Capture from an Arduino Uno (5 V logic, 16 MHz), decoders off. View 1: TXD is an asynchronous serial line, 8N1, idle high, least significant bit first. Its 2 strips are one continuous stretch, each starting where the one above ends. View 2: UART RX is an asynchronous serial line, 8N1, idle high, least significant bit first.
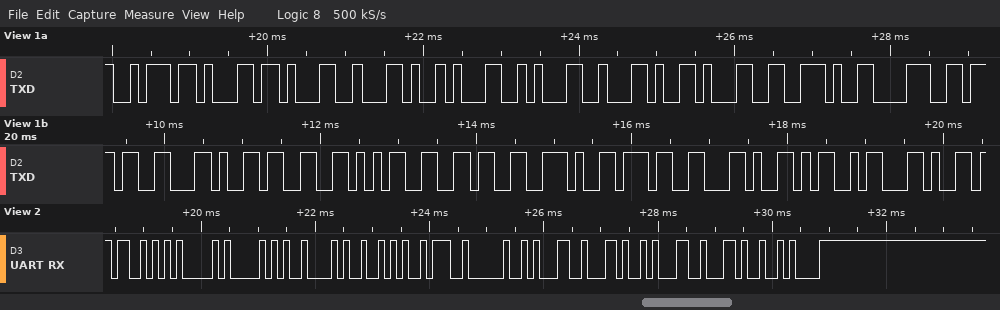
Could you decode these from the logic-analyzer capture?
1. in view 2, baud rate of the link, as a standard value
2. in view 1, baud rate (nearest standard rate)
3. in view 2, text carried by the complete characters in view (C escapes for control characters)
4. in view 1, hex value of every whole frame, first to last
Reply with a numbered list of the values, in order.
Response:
1. 9600 baud
2. 9600 baud
3. "SAPBR: 1,1,\n"
4. 0xBA 0xB1 0x31 0x2C 0x31 0x31 0x2C 0x31 0x2E 0x38 0x37 0x2C 0x33 0x35 0x36 0x2E 0x37 0x2C 0x4D 0x2C
